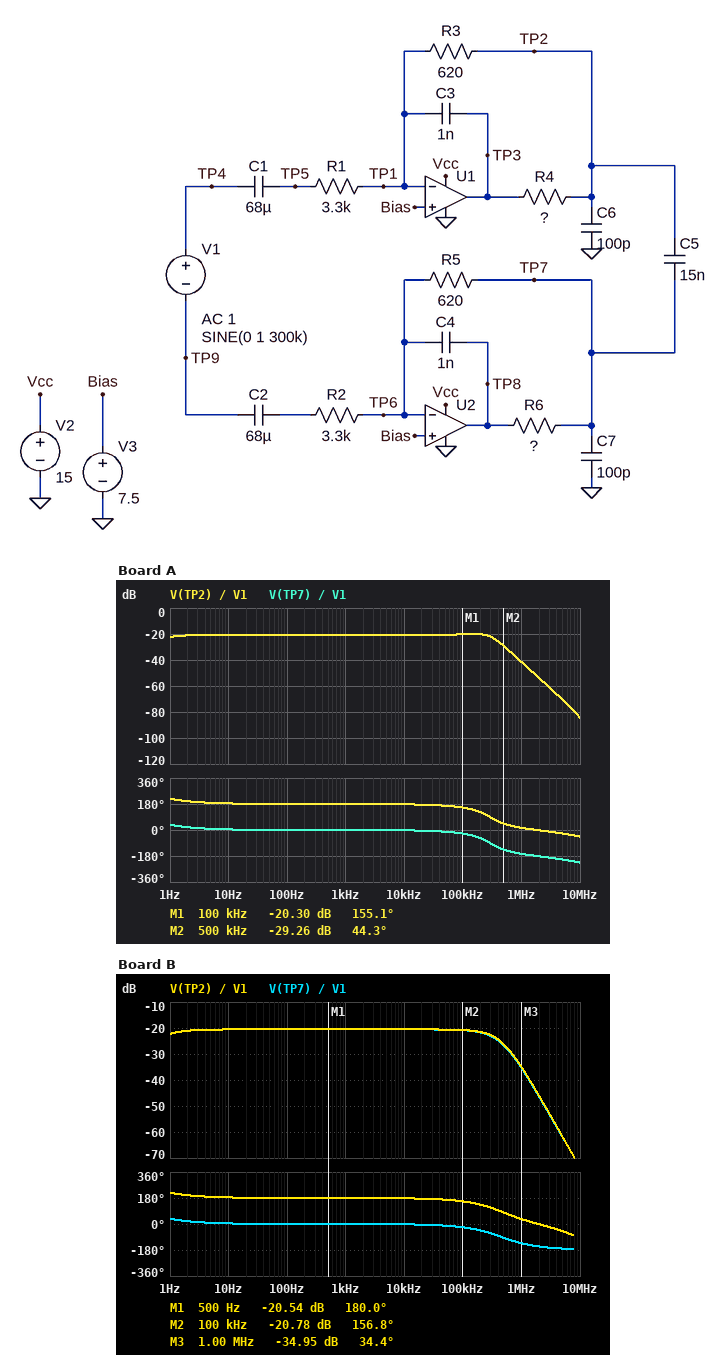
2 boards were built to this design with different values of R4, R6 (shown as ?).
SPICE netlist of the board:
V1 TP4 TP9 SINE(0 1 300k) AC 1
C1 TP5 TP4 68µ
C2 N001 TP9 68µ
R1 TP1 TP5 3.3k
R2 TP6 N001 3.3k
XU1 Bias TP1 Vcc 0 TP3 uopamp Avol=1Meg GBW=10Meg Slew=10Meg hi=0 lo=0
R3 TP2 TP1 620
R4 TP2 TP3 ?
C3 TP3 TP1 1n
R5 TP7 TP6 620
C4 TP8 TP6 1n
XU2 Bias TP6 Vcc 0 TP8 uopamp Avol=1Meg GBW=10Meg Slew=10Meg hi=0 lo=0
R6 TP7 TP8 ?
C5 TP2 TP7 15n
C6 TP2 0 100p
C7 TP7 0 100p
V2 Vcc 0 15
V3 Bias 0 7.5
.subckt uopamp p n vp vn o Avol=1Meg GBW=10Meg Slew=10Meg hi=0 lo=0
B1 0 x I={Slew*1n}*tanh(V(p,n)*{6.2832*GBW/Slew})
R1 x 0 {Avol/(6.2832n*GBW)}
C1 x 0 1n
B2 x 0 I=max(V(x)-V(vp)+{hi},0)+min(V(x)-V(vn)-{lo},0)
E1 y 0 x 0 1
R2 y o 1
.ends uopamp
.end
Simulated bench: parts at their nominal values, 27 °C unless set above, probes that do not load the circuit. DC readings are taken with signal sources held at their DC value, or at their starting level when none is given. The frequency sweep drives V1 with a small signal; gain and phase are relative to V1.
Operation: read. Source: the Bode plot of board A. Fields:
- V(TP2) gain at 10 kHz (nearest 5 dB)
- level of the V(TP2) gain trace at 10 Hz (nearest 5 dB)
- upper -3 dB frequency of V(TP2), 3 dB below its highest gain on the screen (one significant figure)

-20 dB
-20 dB
300 kHz
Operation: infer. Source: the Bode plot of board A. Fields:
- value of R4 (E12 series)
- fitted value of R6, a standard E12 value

15 Ω
15 Ω
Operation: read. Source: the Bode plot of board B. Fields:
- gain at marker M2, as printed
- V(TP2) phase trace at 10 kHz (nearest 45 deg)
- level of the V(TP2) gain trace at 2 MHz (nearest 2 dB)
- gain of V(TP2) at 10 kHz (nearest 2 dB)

-20.78 dB
180 deg
-46 dB
-20 dB
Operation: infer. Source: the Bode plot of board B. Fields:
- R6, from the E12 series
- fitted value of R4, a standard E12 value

5.6 Ω
6.8 Ω
